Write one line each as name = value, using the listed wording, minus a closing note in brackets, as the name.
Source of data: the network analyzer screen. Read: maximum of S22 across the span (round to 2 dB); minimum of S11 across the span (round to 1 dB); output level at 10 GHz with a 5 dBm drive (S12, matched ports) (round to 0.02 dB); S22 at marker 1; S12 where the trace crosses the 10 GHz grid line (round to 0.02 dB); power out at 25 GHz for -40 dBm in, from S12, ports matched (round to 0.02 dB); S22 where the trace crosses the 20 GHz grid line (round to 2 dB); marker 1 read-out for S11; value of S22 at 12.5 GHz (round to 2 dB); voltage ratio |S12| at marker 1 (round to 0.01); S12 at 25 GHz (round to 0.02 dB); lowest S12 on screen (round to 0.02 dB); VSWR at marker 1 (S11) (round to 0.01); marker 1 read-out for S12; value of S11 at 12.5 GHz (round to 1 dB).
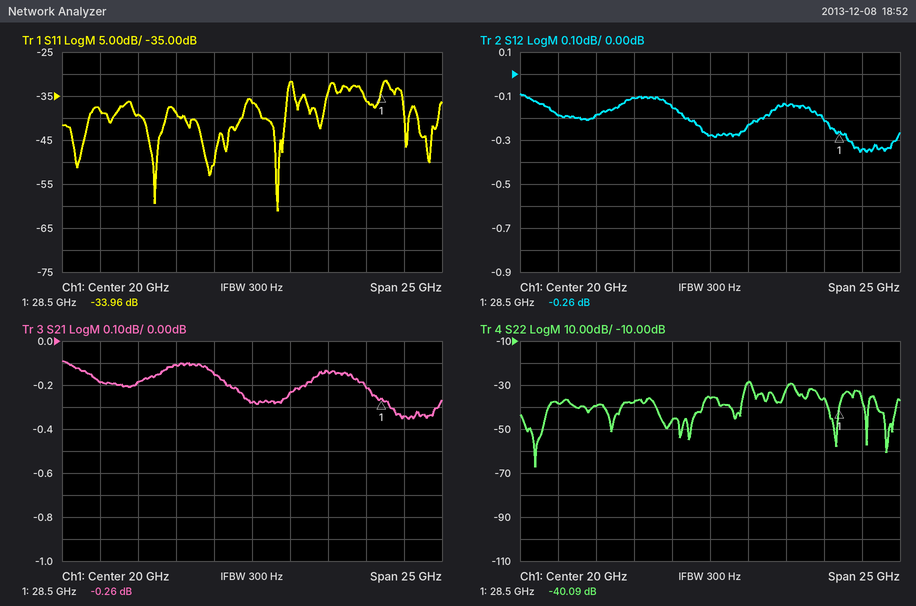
maximum of S22 across the span = -28 dB
minimum of S11 across the span = -61 dB
output level at 10 GHz with a 5 dBm drive (S12, matched ports) = 4.82 dBm
S22 at marker 1 = -40.09 dB
S12 where the trace crosses the 10 GHz grid line = -0.18 dB
power out at 25 GHz for -40 dBm in, from S12, ports matched = -40.14 dBm
S22 where the trace crosses the 20 GHz grid line = -36 dB
marker 1 read-out for S11 = -33.96 dB
value of S22 at 12.5 GHz = -40 dB
voltage ratio |S12| at marker 1 = 0.97
S12 at 25 GHz = -0.14 dB
lowest S12 on screen = -0.36 dB
VSWR at marker 1 (S11) = 1.04
marker 1 read-out for S12 = -0.26 dB
value of S11 at 12.5 GHz = -39 dB
